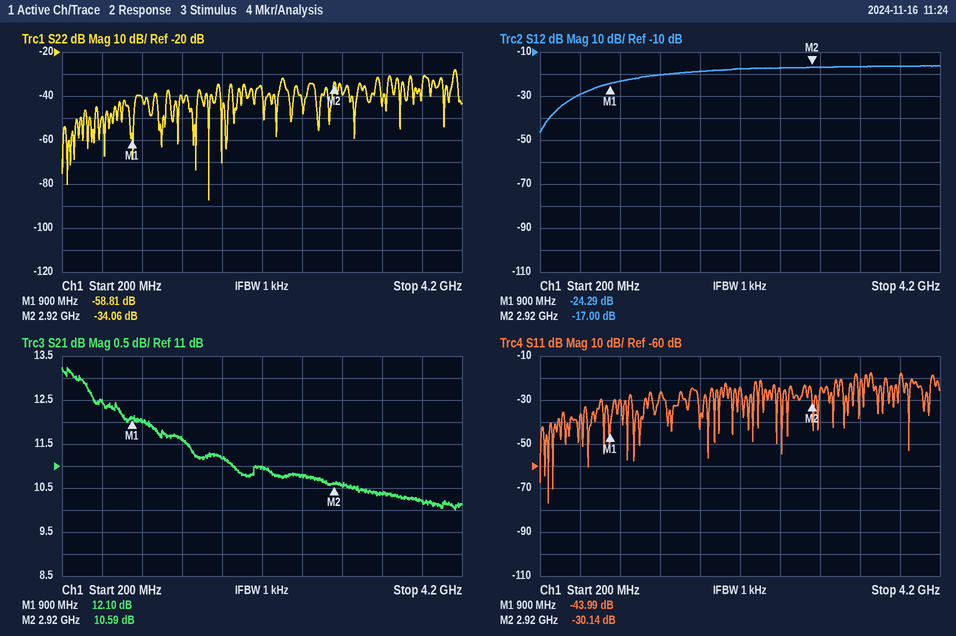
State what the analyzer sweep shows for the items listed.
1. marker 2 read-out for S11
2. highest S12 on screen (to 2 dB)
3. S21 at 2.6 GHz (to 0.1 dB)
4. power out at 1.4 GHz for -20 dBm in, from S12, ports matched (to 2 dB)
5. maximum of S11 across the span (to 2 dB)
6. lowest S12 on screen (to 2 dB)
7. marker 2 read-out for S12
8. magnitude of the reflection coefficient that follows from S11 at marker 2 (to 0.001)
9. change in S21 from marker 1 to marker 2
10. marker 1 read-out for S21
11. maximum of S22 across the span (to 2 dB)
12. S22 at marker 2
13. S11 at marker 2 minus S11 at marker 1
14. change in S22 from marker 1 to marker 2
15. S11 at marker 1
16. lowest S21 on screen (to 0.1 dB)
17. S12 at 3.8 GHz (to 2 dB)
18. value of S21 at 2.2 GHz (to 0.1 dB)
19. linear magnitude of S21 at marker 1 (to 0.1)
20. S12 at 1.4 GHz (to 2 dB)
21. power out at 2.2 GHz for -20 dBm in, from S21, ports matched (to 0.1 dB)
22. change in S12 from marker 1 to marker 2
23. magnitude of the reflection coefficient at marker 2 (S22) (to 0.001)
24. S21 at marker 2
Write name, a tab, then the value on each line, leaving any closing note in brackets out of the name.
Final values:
marker 2 read-out for S11	-30.14 dB
highest S12 on screen	-16 dB
S21 at 2.6 GHz	10.8 dB
power out at 1.4 GHz for -20 dBm in, from S12, ports matched	-40 dBm
maximum of S11 across the span	-18 dB
lowest S12 on screen	-46 dB
marker 2 read-out for S12	-17.00 dB
magnitude of the reflection coefficient that follows from S11 at marker 2	0.031
change in S21 from marker 1 to marker 2	-1.51 dB
marker 1 read-out for S21	12.10 dB
maximum of S22 across the span	-28 dB
S22 at marker 2	-34.06 dB
S11 at marker 2 minus S11 at marker 1	13.85 dB
change in S22 from marker 1 to marker 2	24.75 dB
S11 at marker 1	-43.99 dB
lowest S21 on screen	10.0 dB
S12 at 3.8 GHz	-16 dB
value of S21 at 2.2 GHz	11.0 dB
linear magnitude of S21 at marker 1	4.0
S12 at 1.4 GHz	-20 dB
power out at 2.2 GHz for -20 dBm in, from S21, ports matched	-9.0 dBm
change in S12 from marker 1 to marker 2	7.29 dB
magnitude of the reflection coefficient at marker 2 (S22)	0.020
S21 at marker 2	10.59 dB
